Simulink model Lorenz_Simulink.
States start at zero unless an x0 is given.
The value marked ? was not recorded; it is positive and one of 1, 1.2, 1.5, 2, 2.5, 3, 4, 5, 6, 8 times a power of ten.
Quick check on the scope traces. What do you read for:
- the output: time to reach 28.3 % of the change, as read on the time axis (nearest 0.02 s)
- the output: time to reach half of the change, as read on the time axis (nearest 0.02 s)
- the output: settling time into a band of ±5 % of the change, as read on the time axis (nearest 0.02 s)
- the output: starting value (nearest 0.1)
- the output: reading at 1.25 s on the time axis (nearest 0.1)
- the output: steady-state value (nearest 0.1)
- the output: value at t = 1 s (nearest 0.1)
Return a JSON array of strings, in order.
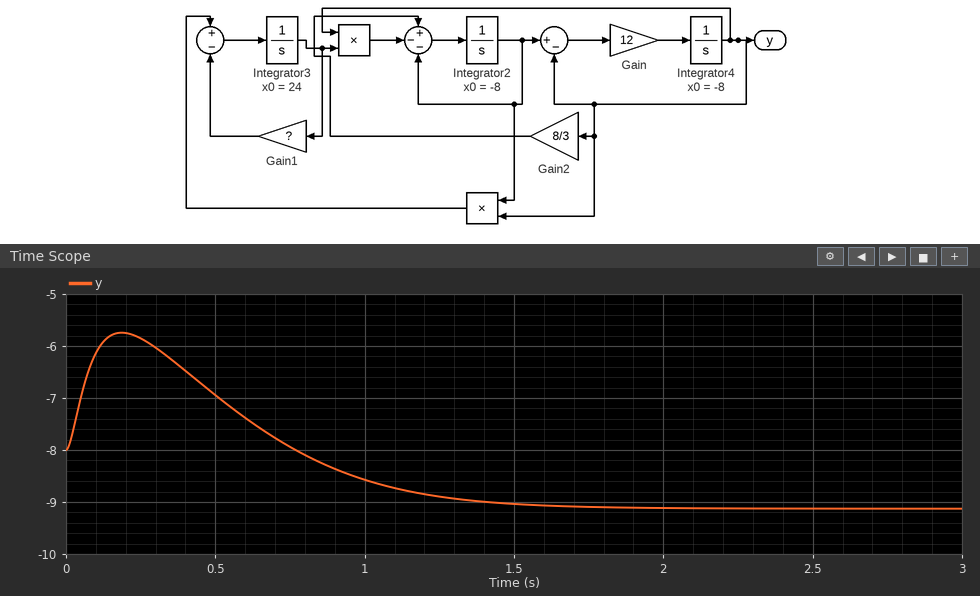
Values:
["0.88 s", "1.00 s", "1.62 s", "-8.0", "-8.9", "-9.1", "-8.6"]
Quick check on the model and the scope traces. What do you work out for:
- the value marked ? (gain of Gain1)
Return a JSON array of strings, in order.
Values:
["50"]
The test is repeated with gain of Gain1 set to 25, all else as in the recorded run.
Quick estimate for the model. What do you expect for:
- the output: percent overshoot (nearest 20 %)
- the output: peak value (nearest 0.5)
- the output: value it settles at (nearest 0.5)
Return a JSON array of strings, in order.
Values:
["220 %", "-3.0", "-6.5"]
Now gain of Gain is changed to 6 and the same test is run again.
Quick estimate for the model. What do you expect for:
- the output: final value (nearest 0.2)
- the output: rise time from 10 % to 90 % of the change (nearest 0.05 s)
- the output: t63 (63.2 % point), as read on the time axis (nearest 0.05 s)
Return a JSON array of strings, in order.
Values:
["-9.2", "0.65 s", "1.20 s"]
